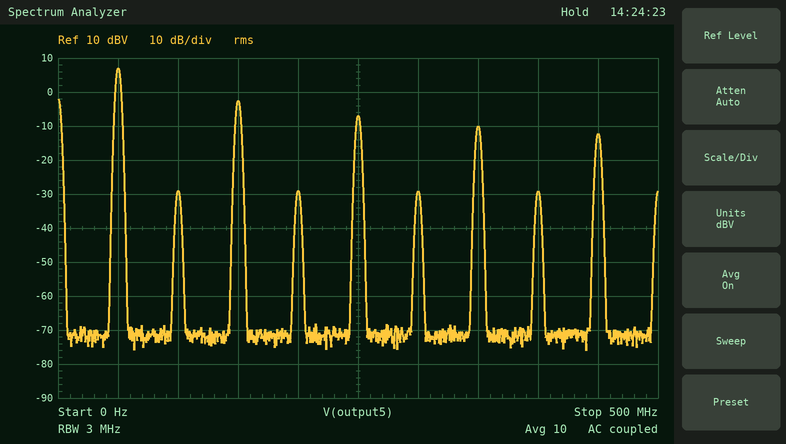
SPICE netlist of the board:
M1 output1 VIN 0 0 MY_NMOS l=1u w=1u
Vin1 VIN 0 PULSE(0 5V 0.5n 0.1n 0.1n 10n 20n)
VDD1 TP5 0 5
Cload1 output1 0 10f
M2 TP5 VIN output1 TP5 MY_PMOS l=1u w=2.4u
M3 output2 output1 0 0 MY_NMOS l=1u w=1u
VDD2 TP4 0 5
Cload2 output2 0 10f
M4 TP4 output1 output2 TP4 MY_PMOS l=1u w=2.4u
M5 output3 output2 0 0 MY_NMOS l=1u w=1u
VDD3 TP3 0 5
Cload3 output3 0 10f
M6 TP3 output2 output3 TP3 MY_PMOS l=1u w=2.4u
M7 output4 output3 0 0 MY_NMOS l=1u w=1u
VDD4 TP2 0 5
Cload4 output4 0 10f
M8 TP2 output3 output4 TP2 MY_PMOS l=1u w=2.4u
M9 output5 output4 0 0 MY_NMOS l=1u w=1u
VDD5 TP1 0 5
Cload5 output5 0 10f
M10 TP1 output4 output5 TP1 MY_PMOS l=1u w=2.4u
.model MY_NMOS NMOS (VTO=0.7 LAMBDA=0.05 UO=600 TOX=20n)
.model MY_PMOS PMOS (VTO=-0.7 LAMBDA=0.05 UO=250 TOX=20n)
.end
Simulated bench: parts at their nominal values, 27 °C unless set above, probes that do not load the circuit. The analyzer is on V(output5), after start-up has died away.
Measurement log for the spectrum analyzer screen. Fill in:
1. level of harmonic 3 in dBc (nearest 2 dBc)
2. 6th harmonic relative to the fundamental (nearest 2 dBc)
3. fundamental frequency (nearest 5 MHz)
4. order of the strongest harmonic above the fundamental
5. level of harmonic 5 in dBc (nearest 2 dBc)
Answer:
-10 dBc
-36 dBc
50 MHz
3
-14 dBc
